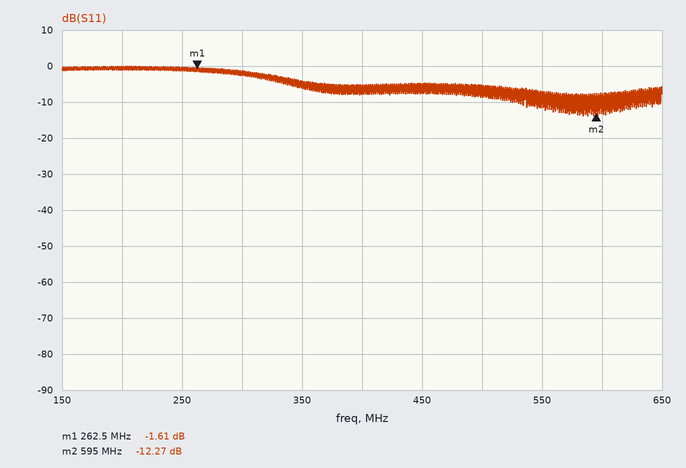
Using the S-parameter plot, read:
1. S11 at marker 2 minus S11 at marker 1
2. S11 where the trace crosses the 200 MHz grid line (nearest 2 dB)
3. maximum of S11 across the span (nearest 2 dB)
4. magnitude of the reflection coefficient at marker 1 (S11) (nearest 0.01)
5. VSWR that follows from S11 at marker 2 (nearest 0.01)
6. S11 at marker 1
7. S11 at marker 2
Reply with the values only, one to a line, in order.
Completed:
-10.66 dB
0 dB
0 dB
0.83
1.64
-1.61 dB
-12.27 dB
